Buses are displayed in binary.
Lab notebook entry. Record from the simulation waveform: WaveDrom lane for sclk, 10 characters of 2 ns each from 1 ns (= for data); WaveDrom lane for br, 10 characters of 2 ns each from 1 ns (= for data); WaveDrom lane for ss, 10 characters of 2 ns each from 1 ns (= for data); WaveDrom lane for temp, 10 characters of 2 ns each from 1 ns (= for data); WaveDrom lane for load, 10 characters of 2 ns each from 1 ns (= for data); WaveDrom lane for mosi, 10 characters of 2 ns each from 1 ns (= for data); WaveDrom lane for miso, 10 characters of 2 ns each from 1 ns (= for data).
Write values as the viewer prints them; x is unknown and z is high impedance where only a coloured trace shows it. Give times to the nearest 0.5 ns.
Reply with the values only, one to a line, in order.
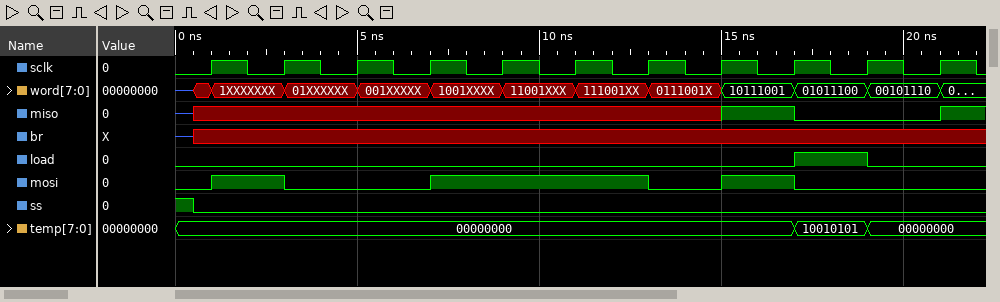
{name: 'sclk', wave: 'p.........'}
{name: 'br', wave: 'x.........'}
{name: 'ss', wave: '0.........'}
{name: 'temp', wave: '=.......==', data: '00000000 10010101 00000000'}
{name: 'load', wave: '0.......10'}
{name: 'mosi', wave: '10.1..010.'}
{name: 'miso', wave: 'x......10.'}
